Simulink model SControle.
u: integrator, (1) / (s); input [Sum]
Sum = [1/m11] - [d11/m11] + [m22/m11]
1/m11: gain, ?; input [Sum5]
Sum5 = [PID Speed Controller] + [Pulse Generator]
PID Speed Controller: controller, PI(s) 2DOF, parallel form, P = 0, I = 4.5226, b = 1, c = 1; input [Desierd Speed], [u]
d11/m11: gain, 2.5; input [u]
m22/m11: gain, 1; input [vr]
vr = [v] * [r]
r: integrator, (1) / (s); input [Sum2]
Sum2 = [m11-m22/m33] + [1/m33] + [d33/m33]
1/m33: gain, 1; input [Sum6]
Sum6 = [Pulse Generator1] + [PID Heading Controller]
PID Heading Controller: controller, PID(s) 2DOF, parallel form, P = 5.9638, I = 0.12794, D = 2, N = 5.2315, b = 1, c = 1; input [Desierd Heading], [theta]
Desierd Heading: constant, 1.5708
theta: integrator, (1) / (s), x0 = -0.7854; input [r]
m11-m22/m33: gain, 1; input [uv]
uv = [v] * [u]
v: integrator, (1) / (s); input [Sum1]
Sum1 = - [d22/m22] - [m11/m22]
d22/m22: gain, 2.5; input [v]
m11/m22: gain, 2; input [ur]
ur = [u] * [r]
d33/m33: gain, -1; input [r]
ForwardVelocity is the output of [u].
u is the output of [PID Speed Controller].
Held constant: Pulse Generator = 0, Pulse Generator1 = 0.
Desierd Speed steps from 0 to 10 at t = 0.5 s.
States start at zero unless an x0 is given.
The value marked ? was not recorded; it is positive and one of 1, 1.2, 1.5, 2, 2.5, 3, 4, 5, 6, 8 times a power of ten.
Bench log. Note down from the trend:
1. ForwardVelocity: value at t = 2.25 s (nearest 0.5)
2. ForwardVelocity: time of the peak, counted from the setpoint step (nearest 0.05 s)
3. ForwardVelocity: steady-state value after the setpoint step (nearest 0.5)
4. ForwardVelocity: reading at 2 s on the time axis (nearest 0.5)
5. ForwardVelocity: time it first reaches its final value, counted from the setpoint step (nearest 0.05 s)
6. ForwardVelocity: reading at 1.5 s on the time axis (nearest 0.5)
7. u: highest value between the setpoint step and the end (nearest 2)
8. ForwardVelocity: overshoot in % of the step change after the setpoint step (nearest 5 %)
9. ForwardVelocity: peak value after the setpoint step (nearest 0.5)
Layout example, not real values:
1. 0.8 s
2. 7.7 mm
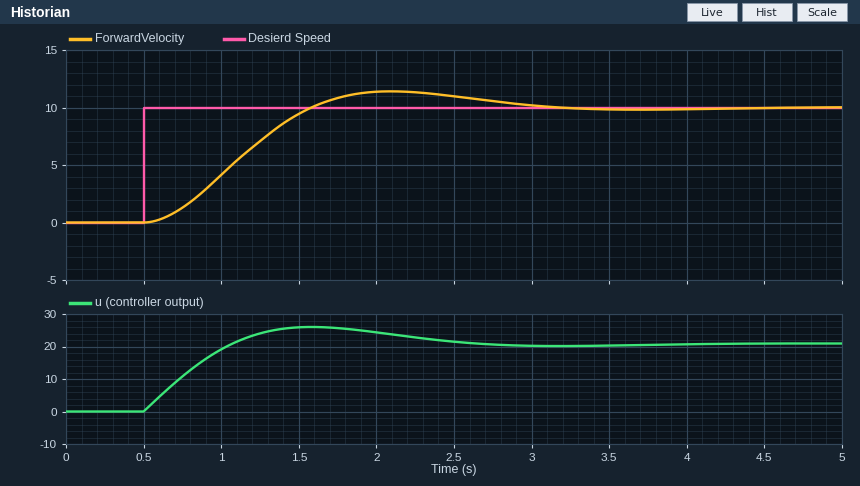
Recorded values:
1. 11.5
2. 1.60 s
3. 10.0
4. 11.5
5. 1.10 s
6. 9.5
7. 26
8. 15 %
9. 11.5
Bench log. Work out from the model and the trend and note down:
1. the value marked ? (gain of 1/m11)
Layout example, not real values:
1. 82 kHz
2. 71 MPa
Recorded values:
1. 1.2
